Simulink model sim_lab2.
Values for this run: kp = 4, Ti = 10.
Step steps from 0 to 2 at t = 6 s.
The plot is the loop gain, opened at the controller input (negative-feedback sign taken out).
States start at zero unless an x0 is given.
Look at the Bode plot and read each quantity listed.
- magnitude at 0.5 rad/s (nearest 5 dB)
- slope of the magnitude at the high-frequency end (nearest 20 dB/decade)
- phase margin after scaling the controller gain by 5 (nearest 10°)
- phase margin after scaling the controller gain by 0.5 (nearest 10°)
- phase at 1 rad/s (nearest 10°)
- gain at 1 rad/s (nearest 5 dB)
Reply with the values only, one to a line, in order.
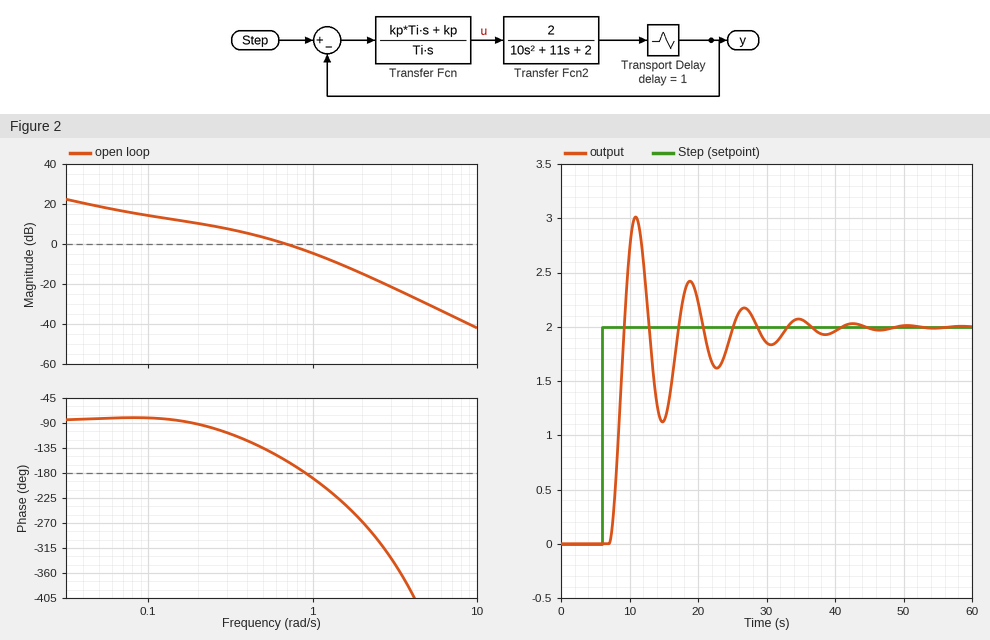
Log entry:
5 dB
-40 dB/decade
-80°
60°
-190°
-5 dB
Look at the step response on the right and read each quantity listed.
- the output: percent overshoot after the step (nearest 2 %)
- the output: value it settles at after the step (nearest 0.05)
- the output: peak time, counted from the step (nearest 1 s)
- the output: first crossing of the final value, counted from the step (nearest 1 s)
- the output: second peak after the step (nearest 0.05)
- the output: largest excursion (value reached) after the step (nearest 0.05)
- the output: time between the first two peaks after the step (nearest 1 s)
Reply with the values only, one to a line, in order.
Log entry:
50 %
2.00
5 s
3 s
2.40
3.00
8 s
